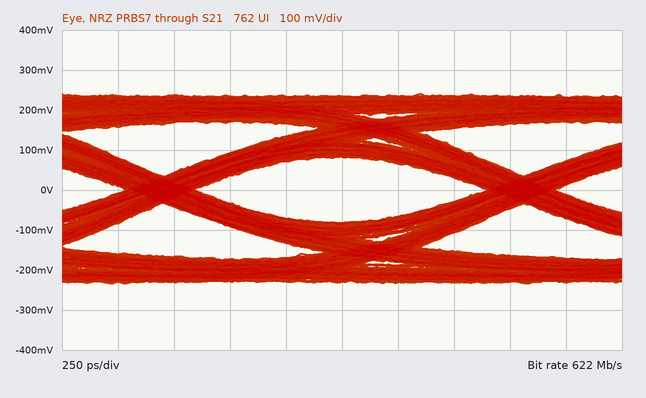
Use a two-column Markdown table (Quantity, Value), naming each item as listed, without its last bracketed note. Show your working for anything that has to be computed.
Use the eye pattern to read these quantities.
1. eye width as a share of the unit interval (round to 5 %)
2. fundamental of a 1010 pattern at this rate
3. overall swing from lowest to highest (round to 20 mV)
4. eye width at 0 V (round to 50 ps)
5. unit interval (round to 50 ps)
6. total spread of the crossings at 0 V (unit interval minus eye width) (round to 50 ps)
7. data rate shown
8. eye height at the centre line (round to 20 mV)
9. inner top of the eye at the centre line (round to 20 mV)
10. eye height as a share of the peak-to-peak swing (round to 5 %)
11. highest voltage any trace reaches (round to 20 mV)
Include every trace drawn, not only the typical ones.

| Quantity | Value |
|---|---|
| eye width as a share of the unit interval | 1.30 ns / 1.60 ns ≈ 81.2 %, so 80 % to the nearest 5 % |
| fundamental of a 1010 pattern at this rate | 311 MHz |
| overall swing from lowest to highest | 480 mV |
| eye width at 0 V | 1.30 ns |
| unit interval | 1.60 ns |
| total spread of the crossings at 0 V (unit interval minus eye width) | 300 ps |
| data rate shown | 622 Mb/s |
| eye height at the centre line | 160 mV |
| inner top of the eye at the centre line | 80 mV |
| eye height as a share of the peak-to-peak swing | 160 mV / 480 mV ≈ 33.3 %, so 35 % to the nearest 5 % |
| highest voltage any trace reaches | 240 mV |
